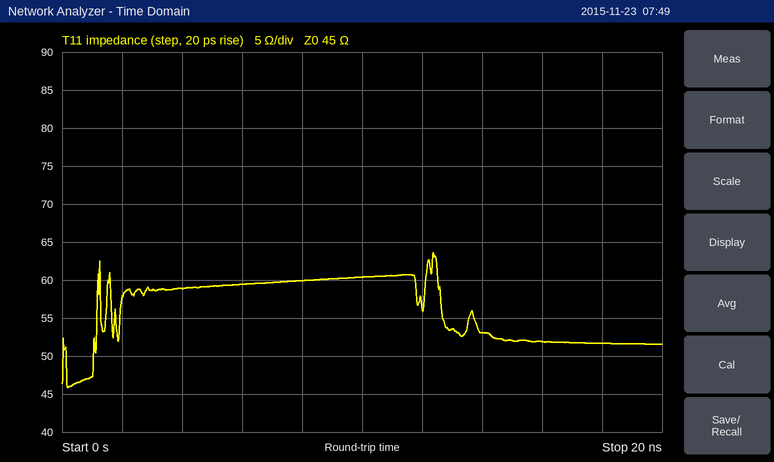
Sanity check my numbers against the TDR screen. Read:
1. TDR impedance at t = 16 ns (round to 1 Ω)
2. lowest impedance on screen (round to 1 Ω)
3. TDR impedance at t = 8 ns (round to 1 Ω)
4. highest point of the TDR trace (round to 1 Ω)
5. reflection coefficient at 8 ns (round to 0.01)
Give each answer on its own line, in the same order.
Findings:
52 Ω
46 Ω
60 Ω
64 Ω
+0.14
